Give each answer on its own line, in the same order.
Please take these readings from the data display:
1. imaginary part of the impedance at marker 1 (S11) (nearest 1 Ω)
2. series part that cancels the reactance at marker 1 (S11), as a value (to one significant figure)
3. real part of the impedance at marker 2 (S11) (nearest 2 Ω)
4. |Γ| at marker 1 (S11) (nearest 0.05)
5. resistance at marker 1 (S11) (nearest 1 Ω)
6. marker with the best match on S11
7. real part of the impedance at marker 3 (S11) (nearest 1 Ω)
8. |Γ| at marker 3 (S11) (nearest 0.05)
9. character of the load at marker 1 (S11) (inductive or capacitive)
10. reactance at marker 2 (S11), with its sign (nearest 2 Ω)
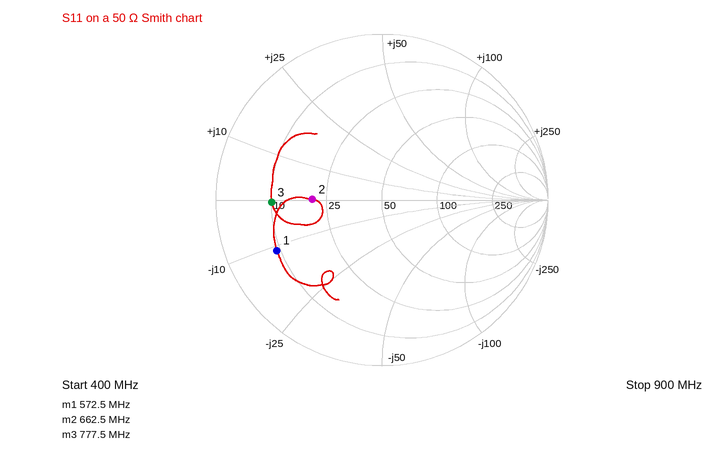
-11 Ω
3 nH
20 Ω
0.70
9 Ω
marker 2
10 Ω
0.65
capacitive
0 Ω
